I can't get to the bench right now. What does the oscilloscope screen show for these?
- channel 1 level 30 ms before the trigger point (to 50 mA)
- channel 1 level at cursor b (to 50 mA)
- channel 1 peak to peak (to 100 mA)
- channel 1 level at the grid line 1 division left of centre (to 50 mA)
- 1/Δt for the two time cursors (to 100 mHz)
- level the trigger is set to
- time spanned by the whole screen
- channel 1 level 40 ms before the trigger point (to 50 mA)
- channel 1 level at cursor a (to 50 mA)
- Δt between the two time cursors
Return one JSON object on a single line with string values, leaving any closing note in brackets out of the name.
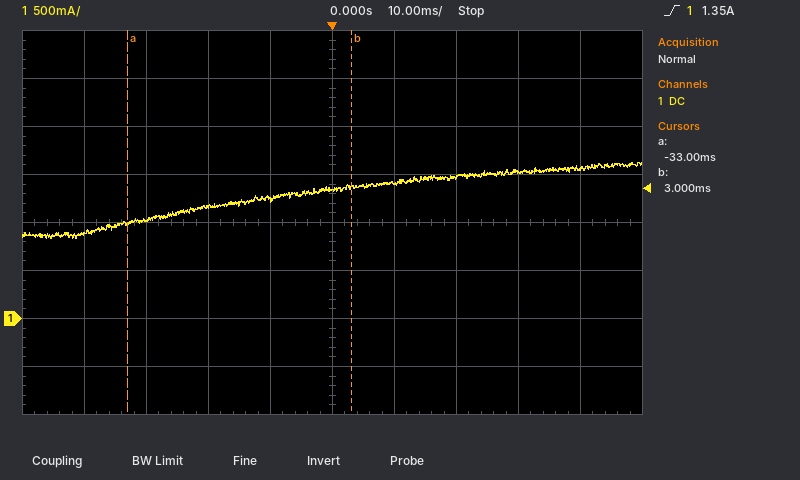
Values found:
{"channel 1 level 30 ms before the trigger point": "1.05 A", "channel 1 level at cursor b": "1.35 A", "channel 1 peak to peak": "800 mA", "channel 1 level at the grid line 1 division left of centre": "1.25 A", "1/Δt for the two time cursors": "27.8 Hz", "level the trigger is set to": "1.35 A", "time spanned by the whole screen": "100 ms", "channel 1 level 40 ms before the trigger point": "900 mA", "channel 1 level at cursor a": "1.00 A", "Δt between the two time cursors": "36 ms"}
